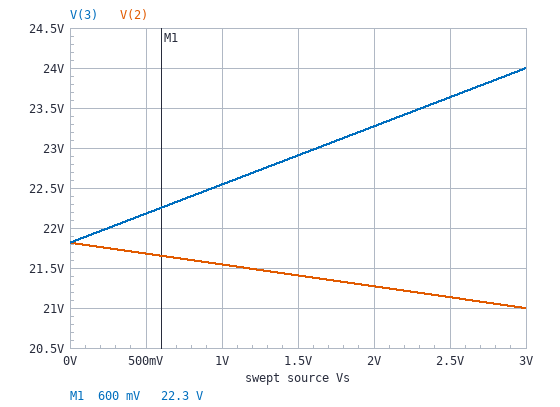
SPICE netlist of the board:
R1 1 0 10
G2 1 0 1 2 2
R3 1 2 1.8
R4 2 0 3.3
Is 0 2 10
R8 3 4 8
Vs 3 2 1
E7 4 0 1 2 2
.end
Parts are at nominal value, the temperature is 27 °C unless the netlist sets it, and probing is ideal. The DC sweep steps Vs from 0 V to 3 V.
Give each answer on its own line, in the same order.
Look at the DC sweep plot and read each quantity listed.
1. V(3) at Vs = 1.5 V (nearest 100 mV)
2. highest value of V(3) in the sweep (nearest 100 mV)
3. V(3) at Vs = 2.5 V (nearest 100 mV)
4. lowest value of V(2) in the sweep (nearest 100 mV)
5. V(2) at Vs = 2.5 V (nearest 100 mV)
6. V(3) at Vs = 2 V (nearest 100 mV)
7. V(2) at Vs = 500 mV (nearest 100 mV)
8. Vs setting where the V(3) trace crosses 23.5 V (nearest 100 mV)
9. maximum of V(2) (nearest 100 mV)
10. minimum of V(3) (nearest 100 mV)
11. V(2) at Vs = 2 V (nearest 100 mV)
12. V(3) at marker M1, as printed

22.9 V
24.0 V
23.6 V
21.0 V
21.1 V
23.3 V
21.7 V
2.3 V
21.8 V
21.8 V
21.3 V
22.3 V
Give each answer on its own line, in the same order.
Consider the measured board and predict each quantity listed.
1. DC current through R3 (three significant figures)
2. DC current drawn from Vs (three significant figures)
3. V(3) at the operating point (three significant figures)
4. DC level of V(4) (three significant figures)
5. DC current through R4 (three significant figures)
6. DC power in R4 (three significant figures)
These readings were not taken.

451 mA
3.02 A
22.5 V
-1.62 V
6.53 A
141 W
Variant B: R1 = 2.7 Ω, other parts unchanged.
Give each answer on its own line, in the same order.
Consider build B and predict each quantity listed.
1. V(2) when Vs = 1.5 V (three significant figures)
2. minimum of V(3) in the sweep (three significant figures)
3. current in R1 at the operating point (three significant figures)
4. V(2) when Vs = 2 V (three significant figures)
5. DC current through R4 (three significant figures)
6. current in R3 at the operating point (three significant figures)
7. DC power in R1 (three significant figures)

18.5 V
18.9 V
6.03 A
18.4 V
5.65 A
1.31 A
98.1 W
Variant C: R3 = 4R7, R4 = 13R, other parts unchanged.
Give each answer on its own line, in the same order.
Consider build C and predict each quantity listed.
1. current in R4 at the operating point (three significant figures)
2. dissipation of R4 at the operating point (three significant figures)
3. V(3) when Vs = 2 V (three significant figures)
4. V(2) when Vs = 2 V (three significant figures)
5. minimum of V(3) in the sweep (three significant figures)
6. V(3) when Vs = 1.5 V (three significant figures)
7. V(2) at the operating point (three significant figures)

3.42 A
152 W
45.9 V
43.9 V
45.1 V
45.7 V
44.5 V
